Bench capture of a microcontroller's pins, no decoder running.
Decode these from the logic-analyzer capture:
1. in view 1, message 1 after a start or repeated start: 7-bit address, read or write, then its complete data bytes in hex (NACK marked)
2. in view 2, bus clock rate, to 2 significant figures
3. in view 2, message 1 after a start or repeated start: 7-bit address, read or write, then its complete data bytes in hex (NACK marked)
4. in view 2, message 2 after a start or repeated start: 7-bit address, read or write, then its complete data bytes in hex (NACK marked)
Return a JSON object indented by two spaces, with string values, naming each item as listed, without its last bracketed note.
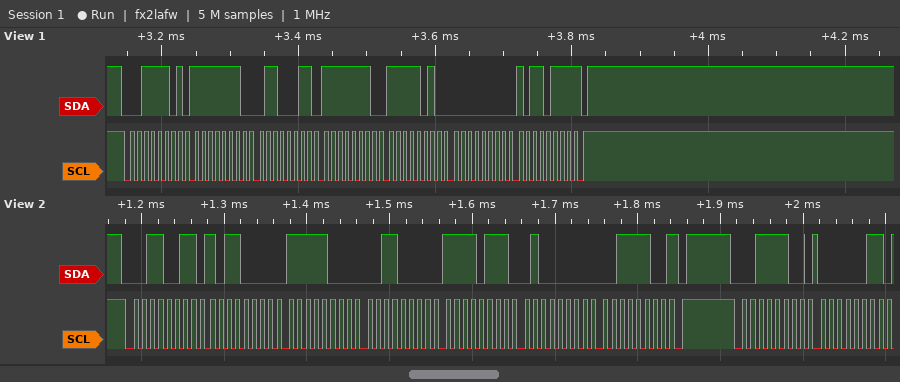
{
  "in view 1, message 1 after a start or repeated start: 7-bit address, read or write, then its complete data bytes in hex": "0x1E read: FE 63 FE FA 00 B7 NACK",
  "in view 2, bus clock rate, to 2 significant figures": "100 kHz",
  "in view 2, message 1 after a start or repeated start: 7-bit address, read or write, then its complete data bytes in hex": "0x19 read: B0 F8 30 F7 40 3C NACK",
  "in view 2, message 2 after a start or repeated start: 7-bit address, read or write, then its complete data bytes in hex": "0x1E write: 03"
}
